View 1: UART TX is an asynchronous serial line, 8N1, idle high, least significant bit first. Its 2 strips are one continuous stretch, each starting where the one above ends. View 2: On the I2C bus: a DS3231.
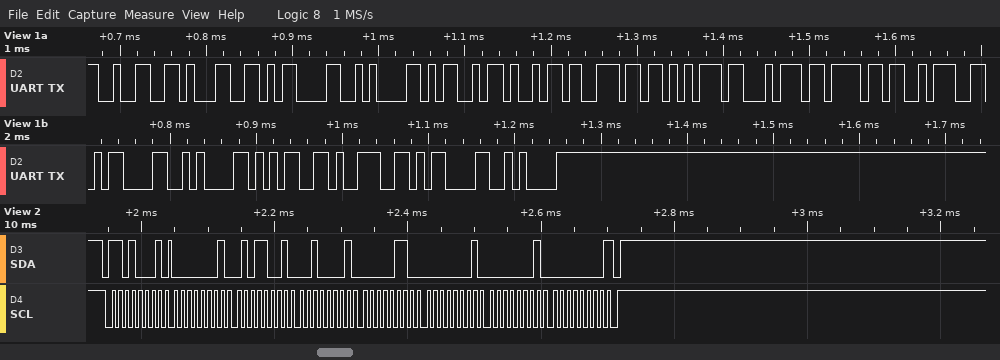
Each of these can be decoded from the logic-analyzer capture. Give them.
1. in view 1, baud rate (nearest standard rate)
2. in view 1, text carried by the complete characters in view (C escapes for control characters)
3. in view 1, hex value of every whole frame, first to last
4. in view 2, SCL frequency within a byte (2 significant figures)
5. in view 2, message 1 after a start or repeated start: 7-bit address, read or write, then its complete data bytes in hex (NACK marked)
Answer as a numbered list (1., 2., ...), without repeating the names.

1. 115200 baud
2. "21\r\nMinuto:\r\n59\r\n"
3. 32 31 0D 0A 4D 69 6E 75 74 6F 3A 0D 0A 35 39 0D 0A
4. 100 kHz
5. 0x68 read: 01 59 21 06 01 01 00 NACK
